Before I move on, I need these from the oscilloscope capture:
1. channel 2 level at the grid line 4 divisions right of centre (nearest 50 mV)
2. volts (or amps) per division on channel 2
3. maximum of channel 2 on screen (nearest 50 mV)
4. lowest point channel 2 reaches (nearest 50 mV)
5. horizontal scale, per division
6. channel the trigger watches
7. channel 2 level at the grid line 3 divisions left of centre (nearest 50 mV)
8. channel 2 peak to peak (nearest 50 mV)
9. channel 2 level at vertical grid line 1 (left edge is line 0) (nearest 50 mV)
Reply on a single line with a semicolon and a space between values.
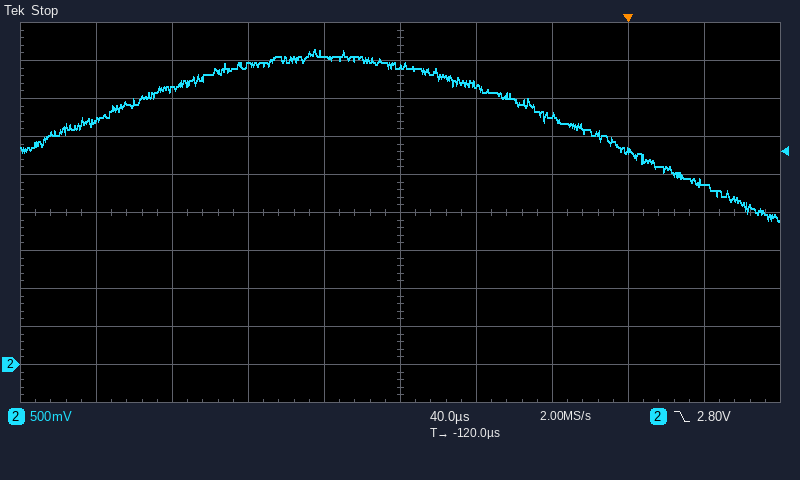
2.40 V; 500 mV; 4.15 V; 1.90 V; 40 µs; channel 2; 3.60 V; 2.25 V; 3.20 V
